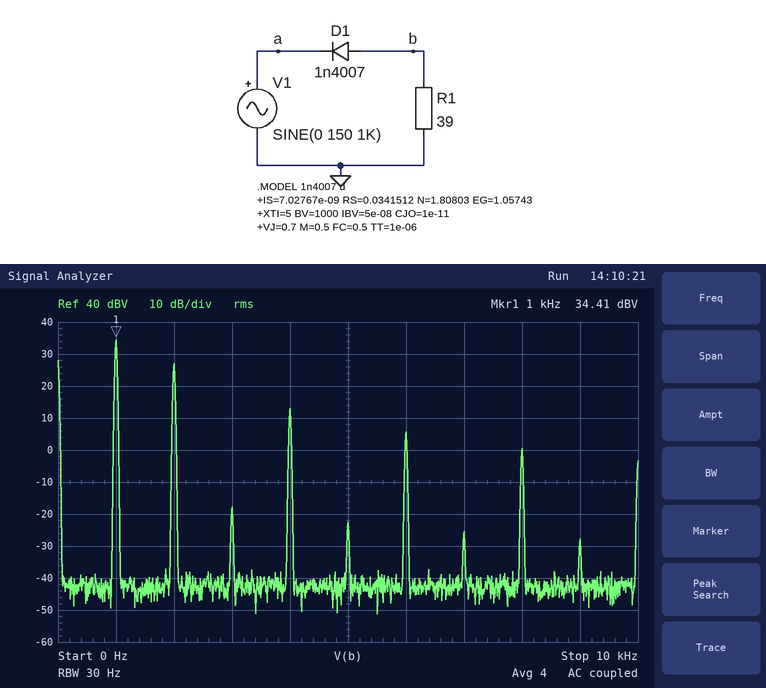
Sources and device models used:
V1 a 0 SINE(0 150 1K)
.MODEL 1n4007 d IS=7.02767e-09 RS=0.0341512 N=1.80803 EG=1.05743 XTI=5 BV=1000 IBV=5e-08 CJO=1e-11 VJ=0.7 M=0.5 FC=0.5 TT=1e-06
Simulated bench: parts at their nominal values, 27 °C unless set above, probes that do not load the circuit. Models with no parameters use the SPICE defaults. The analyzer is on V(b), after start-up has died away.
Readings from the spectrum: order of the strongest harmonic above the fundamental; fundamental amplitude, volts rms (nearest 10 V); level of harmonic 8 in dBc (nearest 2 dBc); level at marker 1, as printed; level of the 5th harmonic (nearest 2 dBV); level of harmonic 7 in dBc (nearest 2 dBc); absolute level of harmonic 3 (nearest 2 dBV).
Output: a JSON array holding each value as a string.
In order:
["2", "50 V", "-34 dBc", "34.41 dBV", "-22 dBV", "-60 dBc", "-18 dBV"]
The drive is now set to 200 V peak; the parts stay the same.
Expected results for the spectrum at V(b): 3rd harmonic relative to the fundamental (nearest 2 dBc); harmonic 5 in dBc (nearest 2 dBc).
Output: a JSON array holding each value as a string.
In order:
["-54 dBc", "-60 dBc"]
